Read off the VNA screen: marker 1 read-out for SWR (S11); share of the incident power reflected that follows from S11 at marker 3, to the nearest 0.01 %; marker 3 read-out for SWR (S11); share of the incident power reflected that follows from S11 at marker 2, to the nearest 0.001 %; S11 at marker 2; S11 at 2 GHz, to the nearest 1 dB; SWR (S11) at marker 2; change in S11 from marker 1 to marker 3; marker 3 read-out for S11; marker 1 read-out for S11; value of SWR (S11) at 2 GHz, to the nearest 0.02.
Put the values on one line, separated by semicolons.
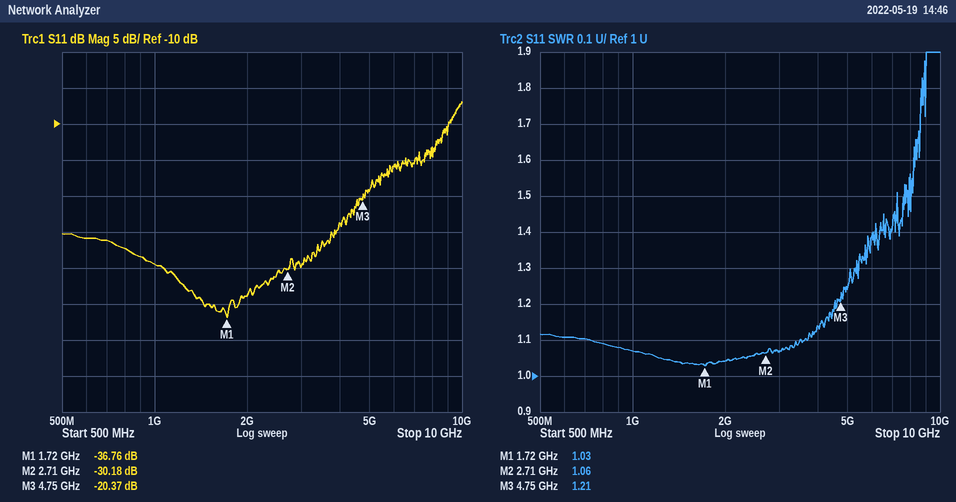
1.03; 0.92 %; 1.21; 0.096 %; -30.18 dB; -34 dB; 1.06; 16.39 dB; -20.37 dB; -36.76 dB; 1.04
